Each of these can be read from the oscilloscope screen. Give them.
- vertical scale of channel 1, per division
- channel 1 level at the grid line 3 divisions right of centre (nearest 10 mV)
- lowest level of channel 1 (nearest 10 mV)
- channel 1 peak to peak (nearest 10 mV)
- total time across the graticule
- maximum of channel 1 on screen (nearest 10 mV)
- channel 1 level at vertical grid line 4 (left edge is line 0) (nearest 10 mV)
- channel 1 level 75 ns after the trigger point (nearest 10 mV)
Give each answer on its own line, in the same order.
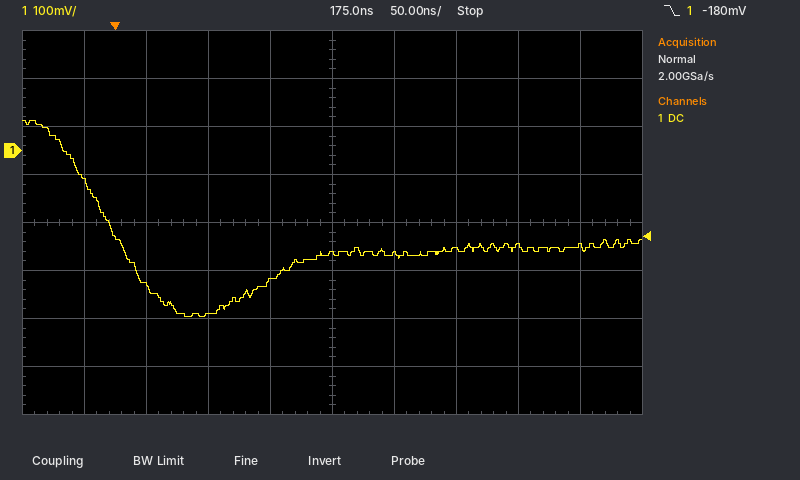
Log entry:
100 mV
-200 mV
-350 mV
410 mV
500 ns
60 mV
-270 mV
-340 mV
